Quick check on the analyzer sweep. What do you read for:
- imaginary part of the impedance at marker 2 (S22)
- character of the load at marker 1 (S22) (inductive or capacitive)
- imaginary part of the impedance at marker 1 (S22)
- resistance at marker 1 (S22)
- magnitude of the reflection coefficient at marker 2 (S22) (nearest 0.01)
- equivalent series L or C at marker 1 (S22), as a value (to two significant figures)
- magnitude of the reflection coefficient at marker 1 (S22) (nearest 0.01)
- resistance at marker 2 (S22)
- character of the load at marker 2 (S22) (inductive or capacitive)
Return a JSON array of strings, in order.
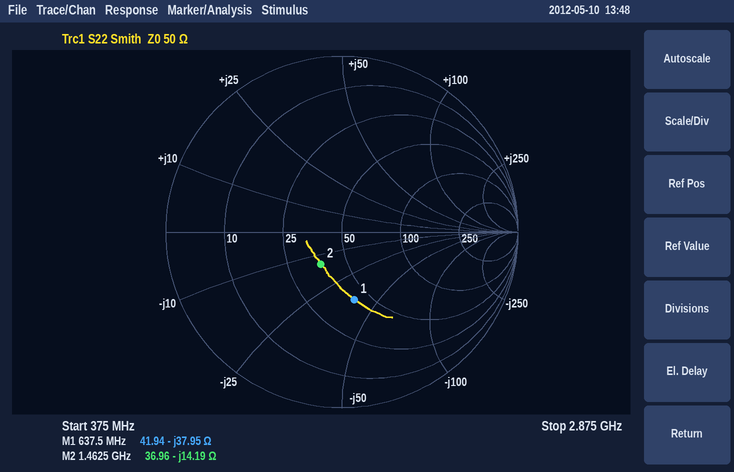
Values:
["-14.19 Ω", "capacitive", "-37.95 Ω", "41.94 Ω", "0.22", "6.6 pF", "0.39", "36.96 Ω", "capacitive"]
